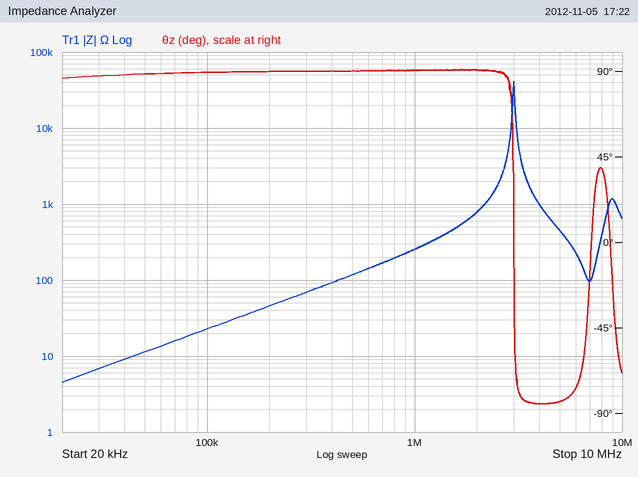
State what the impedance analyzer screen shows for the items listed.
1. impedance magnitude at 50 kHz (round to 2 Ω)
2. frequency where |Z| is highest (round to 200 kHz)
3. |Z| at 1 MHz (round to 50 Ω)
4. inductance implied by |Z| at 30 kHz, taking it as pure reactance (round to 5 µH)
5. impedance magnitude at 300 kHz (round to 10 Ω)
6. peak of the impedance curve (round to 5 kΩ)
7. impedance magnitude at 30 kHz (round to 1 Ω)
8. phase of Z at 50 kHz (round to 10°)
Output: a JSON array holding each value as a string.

["12 Ω", "3.0 MHz", "250 Ω", "35 µH", "70 Ω", "40 kΩ", "7 Ω", "90°"]
